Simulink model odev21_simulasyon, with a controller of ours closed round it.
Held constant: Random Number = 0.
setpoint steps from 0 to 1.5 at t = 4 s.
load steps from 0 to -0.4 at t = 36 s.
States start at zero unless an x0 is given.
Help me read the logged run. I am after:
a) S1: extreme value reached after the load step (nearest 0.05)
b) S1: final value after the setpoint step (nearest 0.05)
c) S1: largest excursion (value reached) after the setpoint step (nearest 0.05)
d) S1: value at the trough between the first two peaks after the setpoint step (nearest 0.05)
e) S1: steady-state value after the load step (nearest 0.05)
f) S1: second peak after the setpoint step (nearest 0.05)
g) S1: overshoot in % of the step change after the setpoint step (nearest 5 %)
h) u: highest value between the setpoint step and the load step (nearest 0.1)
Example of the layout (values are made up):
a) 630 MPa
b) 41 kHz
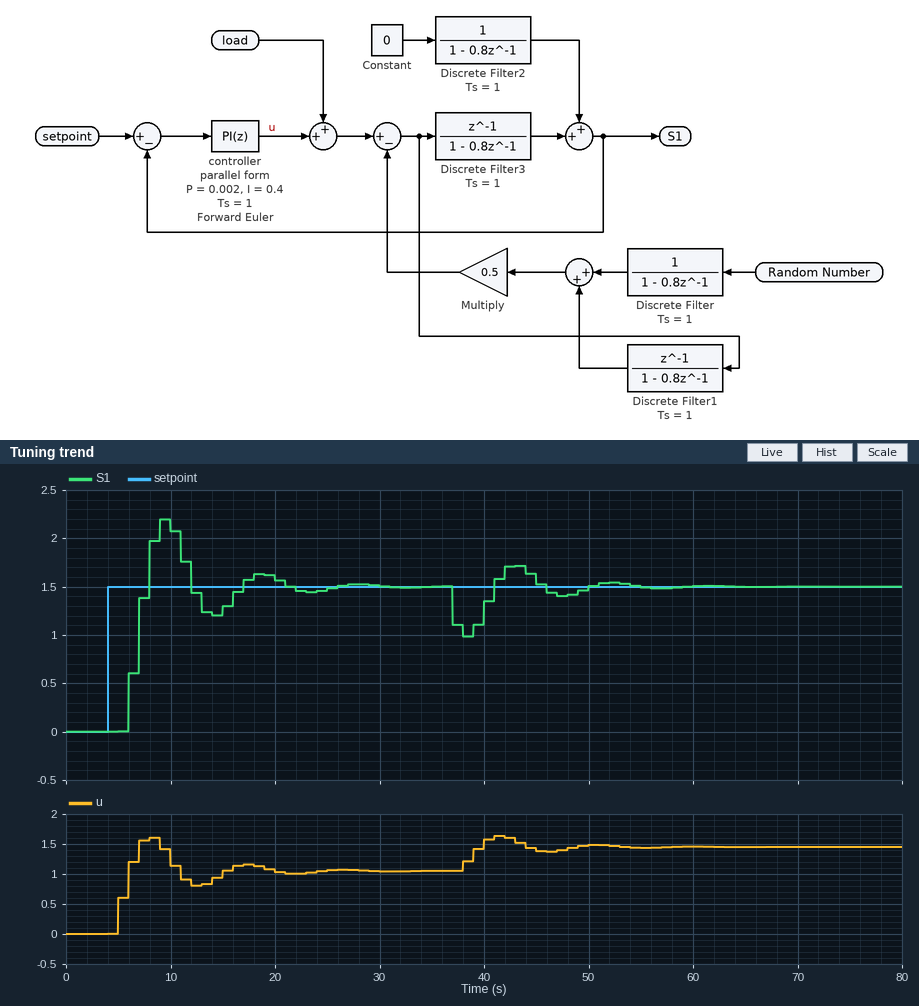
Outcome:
a) 1.00
b) 1.50
c) 2.20
d) 1.20
e) 1.50
f) 1.65
g) 45 %
h) 1.6
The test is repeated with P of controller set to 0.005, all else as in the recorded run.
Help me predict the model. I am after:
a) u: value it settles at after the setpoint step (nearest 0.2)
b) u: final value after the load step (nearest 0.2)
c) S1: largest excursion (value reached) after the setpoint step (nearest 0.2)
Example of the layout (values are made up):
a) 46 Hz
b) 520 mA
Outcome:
a) 1.0
b) 1.4
c) 2.2
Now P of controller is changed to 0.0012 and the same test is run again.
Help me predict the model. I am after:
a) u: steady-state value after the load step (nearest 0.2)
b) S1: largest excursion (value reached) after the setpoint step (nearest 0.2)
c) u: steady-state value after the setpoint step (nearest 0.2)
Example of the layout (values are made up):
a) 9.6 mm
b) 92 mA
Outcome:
a) 1.4
b) 2.2
c) 1.0
